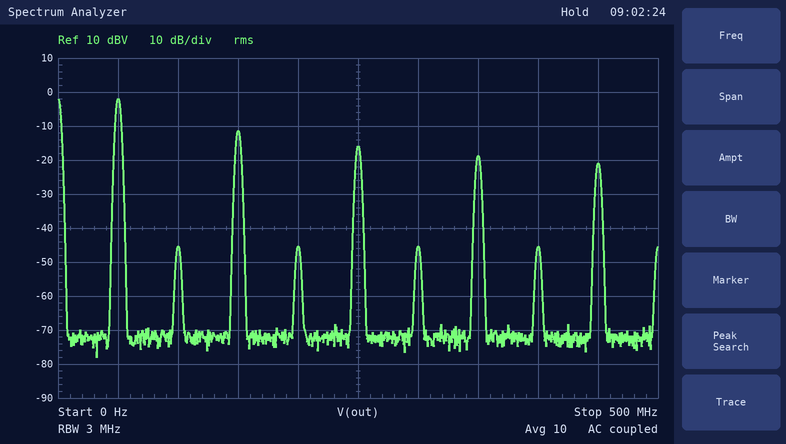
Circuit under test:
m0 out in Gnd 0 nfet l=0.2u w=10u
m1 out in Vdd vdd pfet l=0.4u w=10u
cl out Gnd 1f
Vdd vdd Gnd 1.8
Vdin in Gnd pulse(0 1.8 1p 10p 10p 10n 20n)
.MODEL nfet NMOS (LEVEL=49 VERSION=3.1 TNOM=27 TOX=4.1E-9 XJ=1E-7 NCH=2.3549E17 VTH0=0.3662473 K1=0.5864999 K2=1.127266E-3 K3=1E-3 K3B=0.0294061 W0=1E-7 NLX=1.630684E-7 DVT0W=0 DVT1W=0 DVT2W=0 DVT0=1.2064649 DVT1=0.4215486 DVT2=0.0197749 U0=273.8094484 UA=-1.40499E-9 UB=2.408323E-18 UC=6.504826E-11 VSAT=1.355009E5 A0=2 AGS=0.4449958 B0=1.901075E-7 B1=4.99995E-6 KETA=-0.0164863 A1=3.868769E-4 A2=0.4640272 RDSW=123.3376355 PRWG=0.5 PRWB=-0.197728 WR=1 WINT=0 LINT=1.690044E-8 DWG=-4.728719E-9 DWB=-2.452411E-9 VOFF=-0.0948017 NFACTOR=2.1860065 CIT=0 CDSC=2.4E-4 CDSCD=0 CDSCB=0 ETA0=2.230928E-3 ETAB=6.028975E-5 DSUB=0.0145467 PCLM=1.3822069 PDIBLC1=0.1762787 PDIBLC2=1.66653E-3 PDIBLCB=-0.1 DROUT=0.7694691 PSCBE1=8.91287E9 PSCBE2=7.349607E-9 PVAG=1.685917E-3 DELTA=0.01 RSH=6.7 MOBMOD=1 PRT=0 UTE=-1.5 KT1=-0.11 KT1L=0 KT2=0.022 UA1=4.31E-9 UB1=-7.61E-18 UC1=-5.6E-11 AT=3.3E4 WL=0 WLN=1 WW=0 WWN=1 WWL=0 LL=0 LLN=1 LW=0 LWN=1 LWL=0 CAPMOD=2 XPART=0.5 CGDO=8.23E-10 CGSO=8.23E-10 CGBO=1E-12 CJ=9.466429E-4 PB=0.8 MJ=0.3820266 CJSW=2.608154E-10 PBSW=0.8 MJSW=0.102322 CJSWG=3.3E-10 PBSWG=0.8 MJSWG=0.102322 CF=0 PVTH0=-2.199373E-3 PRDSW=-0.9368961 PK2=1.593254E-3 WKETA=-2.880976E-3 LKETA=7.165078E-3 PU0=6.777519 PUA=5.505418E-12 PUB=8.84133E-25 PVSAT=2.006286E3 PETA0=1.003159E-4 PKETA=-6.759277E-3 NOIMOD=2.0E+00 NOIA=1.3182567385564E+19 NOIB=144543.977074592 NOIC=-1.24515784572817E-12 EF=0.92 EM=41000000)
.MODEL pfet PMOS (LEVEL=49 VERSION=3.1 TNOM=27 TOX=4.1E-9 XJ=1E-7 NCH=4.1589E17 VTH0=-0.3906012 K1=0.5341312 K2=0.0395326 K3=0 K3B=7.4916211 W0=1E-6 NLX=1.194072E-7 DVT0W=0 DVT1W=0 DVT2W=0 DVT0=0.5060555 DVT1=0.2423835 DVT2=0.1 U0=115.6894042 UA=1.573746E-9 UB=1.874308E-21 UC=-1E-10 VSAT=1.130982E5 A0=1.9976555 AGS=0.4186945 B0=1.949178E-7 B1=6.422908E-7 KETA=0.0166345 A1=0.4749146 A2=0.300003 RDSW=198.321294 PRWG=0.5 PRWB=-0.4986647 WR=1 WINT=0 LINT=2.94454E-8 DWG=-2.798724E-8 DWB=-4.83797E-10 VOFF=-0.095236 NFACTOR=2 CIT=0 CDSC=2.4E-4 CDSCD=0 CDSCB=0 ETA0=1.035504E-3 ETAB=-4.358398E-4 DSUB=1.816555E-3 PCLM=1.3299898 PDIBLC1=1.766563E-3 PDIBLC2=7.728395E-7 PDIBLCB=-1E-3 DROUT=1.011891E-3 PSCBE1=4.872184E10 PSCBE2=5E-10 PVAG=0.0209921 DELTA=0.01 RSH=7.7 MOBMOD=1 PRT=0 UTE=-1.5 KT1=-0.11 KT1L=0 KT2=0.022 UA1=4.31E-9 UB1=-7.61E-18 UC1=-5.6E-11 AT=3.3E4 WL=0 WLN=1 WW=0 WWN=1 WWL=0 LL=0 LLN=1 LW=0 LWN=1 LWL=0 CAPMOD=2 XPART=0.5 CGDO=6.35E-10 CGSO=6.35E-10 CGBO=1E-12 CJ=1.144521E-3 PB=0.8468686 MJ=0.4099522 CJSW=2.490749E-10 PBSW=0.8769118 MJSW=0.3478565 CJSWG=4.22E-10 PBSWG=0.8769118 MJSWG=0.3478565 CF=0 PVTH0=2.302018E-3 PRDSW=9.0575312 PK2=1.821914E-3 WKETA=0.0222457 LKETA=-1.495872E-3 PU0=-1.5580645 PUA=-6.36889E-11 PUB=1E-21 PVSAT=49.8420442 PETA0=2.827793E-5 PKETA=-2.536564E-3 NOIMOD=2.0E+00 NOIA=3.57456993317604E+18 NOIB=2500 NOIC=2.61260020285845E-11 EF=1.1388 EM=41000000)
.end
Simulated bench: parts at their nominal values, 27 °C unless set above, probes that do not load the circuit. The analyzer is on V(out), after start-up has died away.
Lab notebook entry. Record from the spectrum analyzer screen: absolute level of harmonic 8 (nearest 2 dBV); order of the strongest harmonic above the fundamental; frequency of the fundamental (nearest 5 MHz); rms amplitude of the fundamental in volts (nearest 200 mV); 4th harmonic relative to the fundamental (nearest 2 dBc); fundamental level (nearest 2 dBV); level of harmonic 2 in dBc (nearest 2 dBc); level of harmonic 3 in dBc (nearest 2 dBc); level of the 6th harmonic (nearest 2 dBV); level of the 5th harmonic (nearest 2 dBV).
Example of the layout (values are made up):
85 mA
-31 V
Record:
-46 dBV
3
50 MHz
800 mV
-44 dBc
-2 dBV
-44 dBc
-10 dBc
-46 dBV
-16 dBV
